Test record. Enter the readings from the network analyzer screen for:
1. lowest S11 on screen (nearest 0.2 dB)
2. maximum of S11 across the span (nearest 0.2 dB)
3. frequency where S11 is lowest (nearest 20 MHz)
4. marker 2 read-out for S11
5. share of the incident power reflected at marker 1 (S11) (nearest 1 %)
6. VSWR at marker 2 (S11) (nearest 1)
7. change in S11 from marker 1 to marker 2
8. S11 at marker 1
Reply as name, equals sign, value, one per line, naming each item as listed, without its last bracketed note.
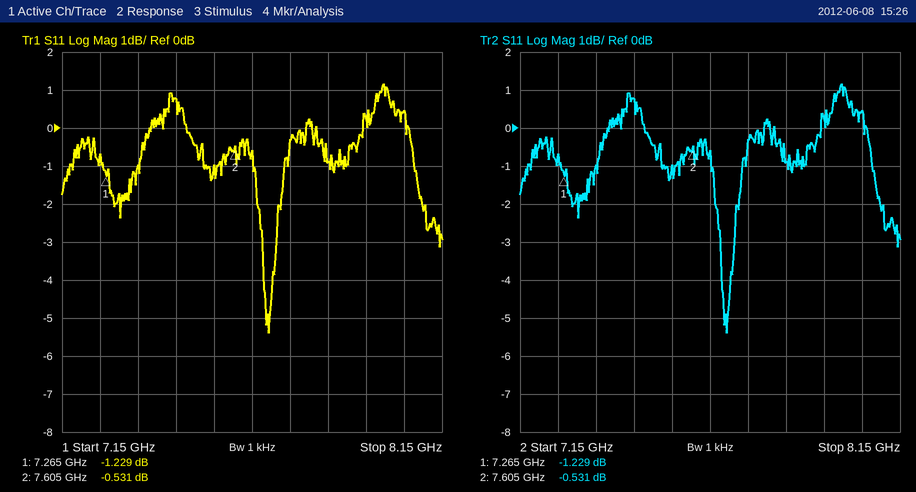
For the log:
lowest S11 on screen = -5.4 dB
maximum of S11 across the span = 1.2 dB
frequency where S11 is lowest = 7.70 GHz
marker 2 read-out for S11 = -0.531 dB
share of the incident power reflected at marker 1 (S11) = 75 %
VSWR at marker 2 (S11) = 33
change in S11 from marker 1 to marker 2 = 0.698 dB
S11 at marker 1 = -1.229 dB
